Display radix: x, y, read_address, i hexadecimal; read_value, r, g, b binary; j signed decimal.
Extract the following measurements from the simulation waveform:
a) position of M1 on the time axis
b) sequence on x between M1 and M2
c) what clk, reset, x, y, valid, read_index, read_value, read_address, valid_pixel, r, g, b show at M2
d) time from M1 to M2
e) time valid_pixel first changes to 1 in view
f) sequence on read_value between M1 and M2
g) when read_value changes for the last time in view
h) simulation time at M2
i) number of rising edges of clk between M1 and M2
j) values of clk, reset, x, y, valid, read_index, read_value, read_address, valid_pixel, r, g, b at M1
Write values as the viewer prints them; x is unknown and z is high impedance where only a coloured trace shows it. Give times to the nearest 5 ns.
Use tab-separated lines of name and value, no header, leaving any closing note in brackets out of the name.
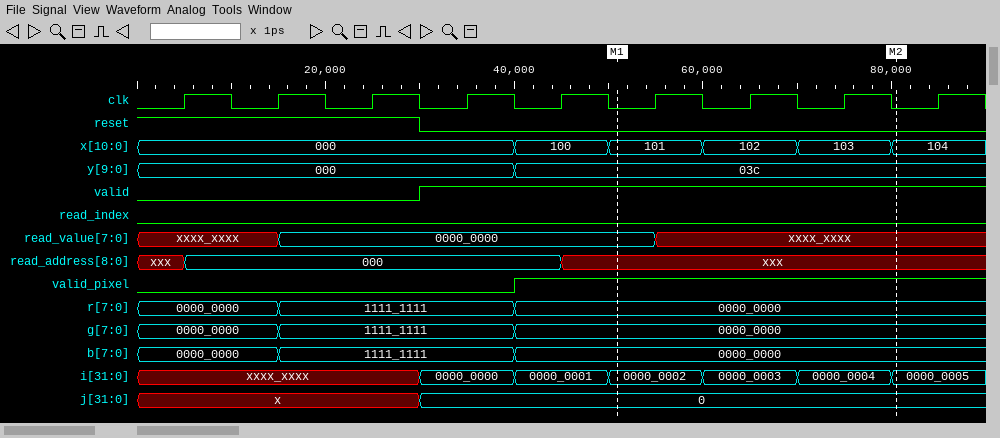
position of M1 on the time axis	50 ns
sequence on x between M1 and M2	101, 102, 103, 104
what clk, reset, x, y, valid, read_index, read_value, read_address, valid_pixel, r, g, b show at M2	clk=0, reset=0, x=104, y=03c, valid=1, read_index=0, read_value=xxxx_xxxx, read_address=xxx, valid_pixel=1, r=0000_0000, g=0000_0000, b=0000_0000
time from M1 to M2	30 ns
time valid_pixel first changes to 1 in view	40 ns
sequence on read_value between M1 and M2	0000_0000, xxxx_xxxx
when read_value changes for the last time in view	55 ns
simulation time at M2	80 ns
number of rising edges of clk between M1 and M2	3
values of clk, reset, x, y, valid, read_index, read_value, read_address, valid_pixel, r, g, b at M1	clk=0, reset=0, x=101, y=03c, valid=1, read_index=0, read_value=0000_0000, read_address=xxx, valid_pixel=1, r=0000_0000, g=0000_0000, b=0000_0000
